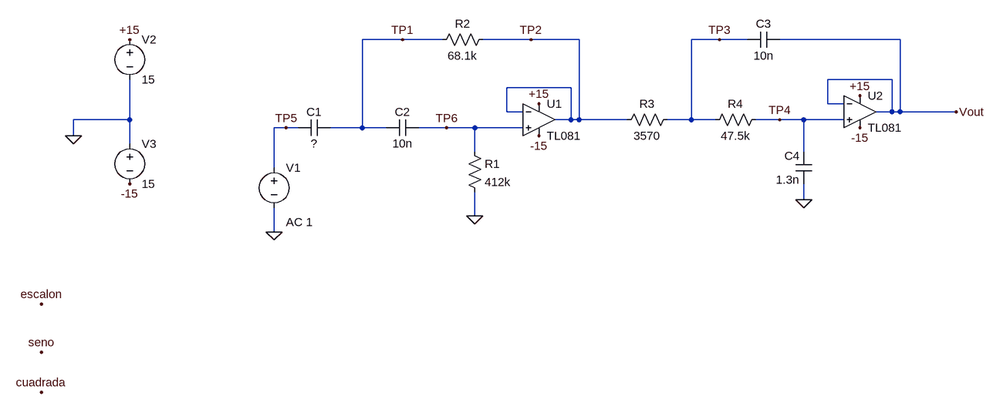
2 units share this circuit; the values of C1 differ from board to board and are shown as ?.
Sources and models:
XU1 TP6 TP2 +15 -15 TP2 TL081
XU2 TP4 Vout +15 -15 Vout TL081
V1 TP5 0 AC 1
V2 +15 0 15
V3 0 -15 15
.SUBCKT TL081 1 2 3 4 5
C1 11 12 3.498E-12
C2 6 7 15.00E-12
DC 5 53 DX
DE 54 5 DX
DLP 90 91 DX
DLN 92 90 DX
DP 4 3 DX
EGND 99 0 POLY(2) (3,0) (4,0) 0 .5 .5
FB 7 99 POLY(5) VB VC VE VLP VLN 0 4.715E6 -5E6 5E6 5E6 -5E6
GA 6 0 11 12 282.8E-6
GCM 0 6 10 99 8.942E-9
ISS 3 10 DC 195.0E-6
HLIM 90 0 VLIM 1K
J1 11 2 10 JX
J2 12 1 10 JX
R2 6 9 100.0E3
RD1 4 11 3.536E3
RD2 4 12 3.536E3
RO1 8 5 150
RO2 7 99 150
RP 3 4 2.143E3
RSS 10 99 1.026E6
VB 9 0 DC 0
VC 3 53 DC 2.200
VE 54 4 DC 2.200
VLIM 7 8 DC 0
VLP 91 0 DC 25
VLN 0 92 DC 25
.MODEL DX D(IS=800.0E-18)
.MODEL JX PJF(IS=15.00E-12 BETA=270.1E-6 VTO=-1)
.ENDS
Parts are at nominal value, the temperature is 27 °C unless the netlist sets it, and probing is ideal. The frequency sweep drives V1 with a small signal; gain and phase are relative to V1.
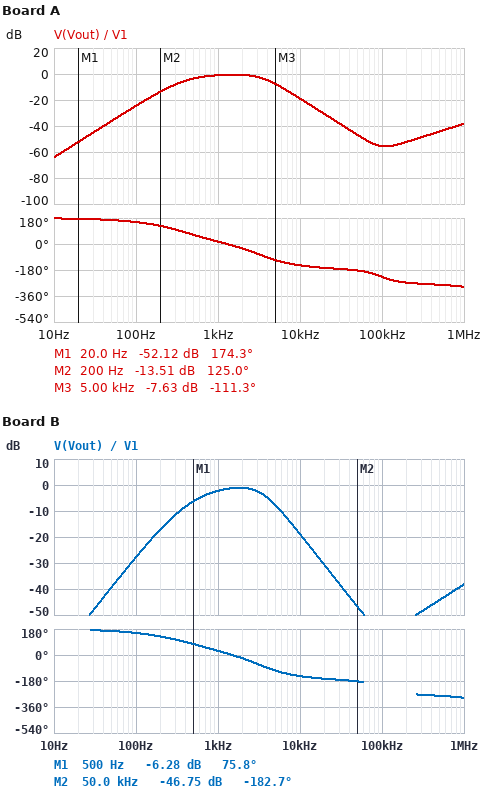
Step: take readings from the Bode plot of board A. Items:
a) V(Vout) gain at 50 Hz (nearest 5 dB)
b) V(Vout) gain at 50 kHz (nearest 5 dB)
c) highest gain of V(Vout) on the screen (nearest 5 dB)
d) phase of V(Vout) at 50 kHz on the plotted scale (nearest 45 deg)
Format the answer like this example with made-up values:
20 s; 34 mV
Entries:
-35 dB; -45 dB; 0 dB; -180 deg
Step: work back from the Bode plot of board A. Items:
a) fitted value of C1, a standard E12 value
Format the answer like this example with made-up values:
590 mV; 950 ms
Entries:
560 pF
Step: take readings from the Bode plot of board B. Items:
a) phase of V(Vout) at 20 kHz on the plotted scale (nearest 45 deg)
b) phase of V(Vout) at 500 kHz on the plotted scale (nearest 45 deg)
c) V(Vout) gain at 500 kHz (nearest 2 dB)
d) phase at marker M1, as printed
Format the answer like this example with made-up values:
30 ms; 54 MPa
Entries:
-180 deg; -270 deg; -44 dB; 75.8 deg
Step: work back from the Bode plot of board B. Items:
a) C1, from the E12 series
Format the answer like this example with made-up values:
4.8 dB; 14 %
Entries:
390 pF
